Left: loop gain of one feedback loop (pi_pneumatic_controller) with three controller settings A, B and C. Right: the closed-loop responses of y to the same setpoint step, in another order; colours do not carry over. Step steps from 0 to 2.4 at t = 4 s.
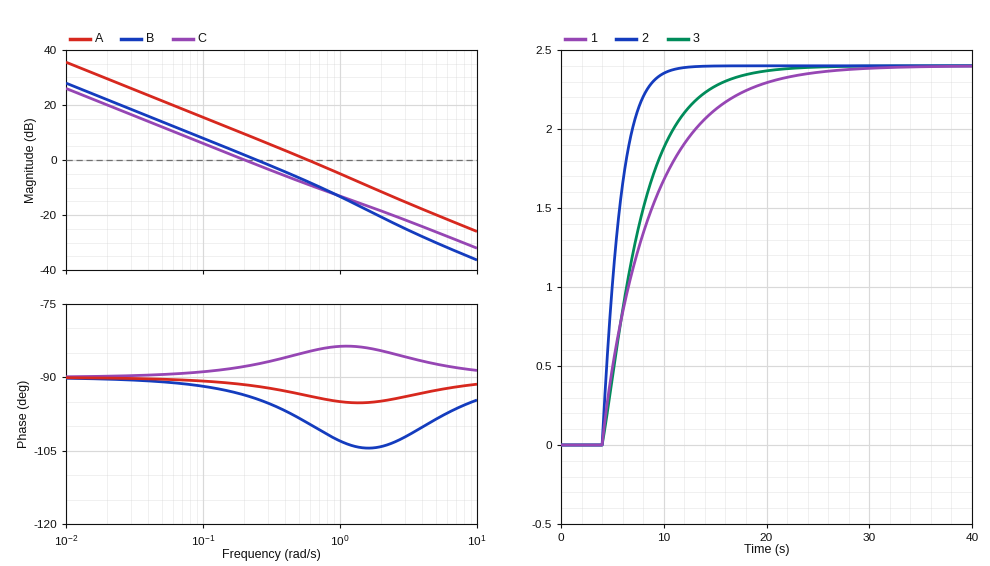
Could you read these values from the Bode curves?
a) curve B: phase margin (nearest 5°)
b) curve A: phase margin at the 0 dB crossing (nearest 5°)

85°
85°
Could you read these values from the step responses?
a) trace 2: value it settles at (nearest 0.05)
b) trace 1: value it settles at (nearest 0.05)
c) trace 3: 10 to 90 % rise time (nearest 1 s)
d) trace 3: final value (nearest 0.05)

2.40
2.40
8 s
2.40
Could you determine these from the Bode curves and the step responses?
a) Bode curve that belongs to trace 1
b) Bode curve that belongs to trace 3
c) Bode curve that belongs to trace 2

C
B
A
